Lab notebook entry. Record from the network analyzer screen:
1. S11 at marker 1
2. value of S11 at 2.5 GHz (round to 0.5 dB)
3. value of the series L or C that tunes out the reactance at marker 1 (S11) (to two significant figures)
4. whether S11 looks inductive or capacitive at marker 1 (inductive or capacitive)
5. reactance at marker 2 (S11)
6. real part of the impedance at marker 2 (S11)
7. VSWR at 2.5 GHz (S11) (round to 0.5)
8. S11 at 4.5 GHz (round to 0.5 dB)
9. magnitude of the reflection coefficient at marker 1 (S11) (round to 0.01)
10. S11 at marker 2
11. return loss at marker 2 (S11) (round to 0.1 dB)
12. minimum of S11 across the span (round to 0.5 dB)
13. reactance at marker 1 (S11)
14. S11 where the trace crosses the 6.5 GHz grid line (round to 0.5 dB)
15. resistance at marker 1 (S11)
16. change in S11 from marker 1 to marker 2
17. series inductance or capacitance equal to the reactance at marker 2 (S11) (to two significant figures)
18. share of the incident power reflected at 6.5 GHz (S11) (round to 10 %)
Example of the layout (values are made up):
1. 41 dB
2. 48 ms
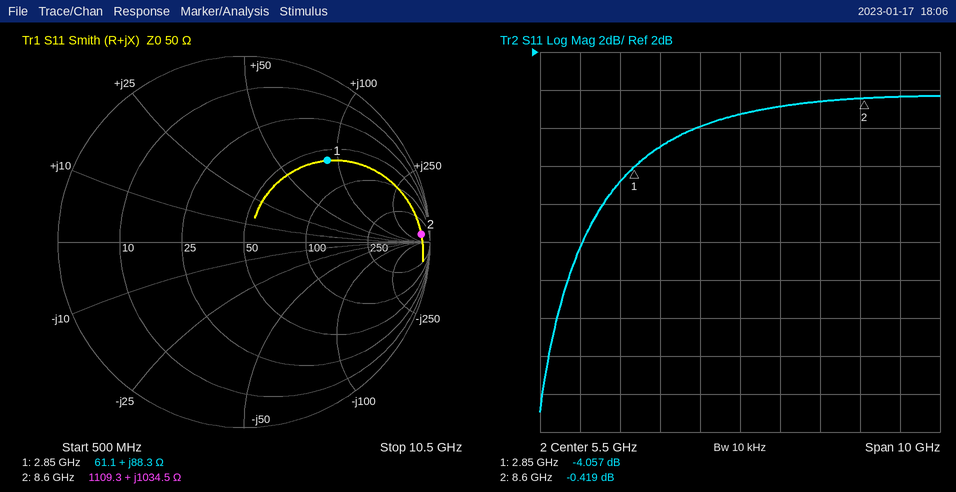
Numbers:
1. -4.057 dB
2. -5.0 dB
3. 630 fF
4. inductive
5. +1034.5 Ω
6. 1109.3 Ω
7. 3.5
8. -2.0 dB
9. 0.63
10. -0.419 dB
11. 0.4 dB
12. -17.0 dB
13. +88.3 Ω
14. -1.0 dB
15. 61.1 Ω
16. 3.638 dB
17. 19 nH
18. 80 %
